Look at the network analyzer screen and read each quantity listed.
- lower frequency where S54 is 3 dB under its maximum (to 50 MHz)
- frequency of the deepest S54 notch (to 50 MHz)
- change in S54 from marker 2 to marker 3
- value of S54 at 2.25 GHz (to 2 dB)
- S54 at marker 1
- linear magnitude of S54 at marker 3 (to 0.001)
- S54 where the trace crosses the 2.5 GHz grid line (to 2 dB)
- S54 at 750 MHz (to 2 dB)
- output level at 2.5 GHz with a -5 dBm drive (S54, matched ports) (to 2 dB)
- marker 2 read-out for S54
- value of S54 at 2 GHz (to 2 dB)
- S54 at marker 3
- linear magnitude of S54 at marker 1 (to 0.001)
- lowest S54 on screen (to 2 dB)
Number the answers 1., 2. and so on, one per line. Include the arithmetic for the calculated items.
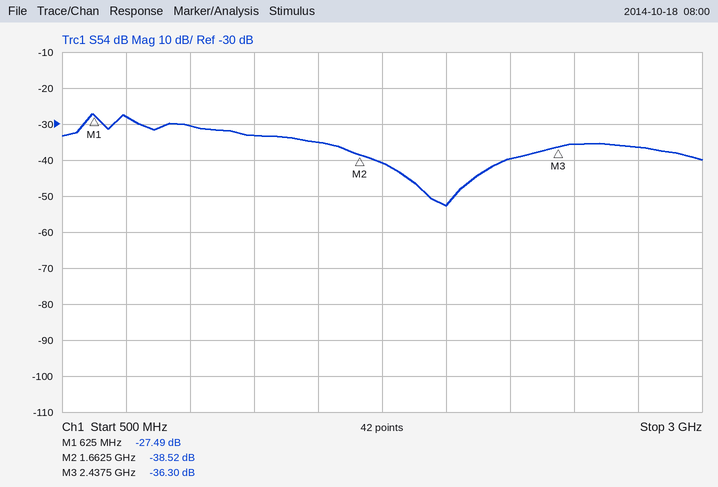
1. 600 MHz
2. 2.00 GHz
3. -36.3 − (-38.52) = 2.22 dB
4. -40 dB
5. -27.49 dB
6. 10^(-36.3/20) ≈ 0.015
7. -36 dB
8. -28 dB
9. -5 dBm + (-36 dB) = -40 dBm
10. -38.52 dB
11. -52 dB
12. -36.30 dB
13. 10^(-27.49/20) ≈ 0.042
14. -52 dB
